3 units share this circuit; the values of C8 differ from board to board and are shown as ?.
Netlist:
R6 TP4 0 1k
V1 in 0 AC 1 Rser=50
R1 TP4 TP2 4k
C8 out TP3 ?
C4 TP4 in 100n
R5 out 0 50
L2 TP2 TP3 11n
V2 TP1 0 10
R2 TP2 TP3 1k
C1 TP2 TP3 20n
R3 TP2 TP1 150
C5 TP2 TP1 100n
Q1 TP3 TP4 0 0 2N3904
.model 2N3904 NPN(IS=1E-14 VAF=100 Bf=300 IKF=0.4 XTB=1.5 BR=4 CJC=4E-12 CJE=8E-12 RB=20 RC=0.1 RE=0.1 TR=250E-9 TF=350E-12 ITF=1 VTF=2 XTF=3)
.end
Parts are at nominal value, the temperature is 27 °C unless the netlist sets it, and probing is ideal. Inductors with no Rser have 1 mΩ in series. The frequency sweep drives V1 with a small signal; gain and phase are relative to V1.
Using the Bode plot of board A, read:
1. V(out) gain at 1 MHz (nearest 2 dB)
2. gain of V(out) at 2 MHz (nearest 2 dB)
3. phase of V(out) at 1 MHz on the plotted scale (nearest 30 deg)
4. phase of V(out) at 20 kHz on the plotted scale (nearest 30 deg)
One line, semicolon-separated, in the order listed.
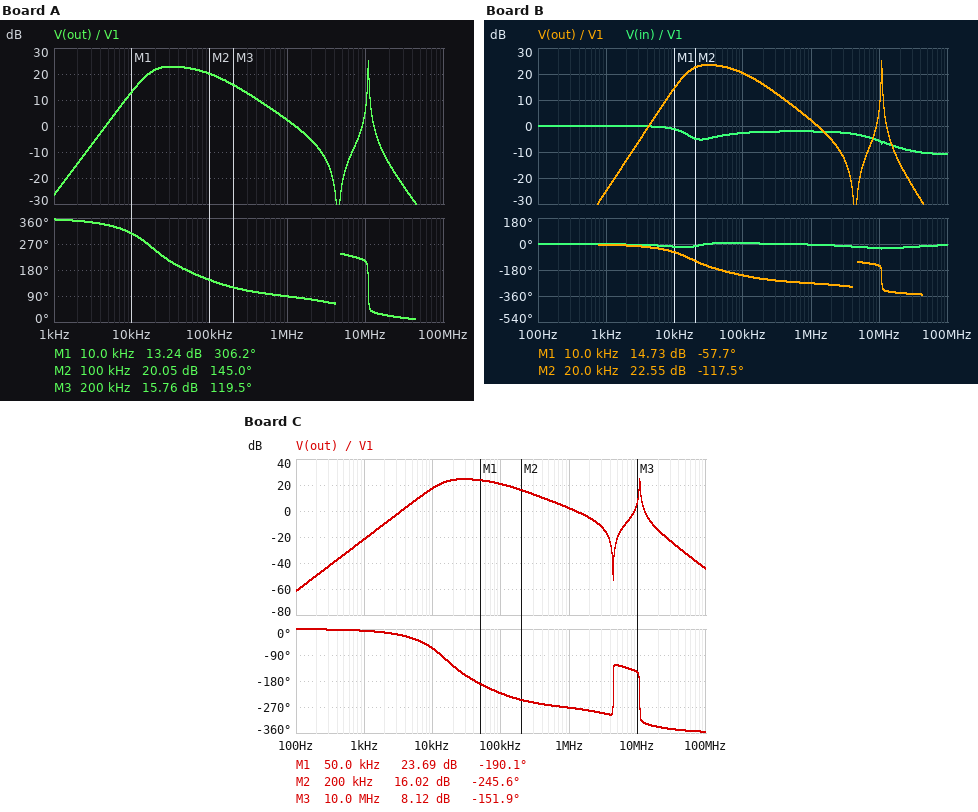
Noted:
2 dB; -6 dB; 90 deg; 240 deg
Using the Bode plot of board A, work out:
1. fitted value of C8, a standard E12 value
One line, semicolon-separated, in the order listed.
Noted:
68 nF
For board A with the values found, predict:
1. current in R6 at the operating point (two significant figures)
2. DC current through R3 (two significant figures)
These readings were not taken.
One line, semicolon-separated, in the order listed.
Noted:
760 µA; 38 mA
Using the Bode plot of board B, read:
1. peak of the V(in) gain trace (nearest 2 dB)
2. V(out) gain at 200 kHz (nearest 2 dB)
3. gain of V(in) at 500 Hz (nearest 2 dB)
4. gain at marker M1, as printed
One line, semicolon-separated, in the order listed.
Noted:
0 dB; 16 dB; 0 dB; 14.73 dB
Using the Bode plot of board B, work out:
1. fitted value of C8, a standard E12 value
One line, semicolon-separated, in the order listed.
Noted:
82 nF
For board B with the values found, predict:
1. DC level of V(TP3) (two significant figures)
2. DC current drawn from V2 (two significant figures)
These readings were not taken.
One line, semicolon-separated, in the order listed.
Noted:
4.3 V; 38 mA
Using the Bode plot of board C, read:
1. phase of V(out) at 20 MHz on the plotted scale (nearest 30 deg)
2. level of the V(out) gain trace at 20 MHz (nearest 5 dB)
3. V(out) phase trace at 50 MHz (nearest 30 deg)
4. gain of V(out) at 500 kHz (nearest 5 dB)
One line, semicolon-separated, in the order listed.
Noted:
-330 deg; -15 dB; -360 deg; 10 dB
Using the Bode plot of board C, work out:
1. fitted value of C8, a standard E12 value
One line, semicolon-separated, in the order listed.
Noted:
120 nF
